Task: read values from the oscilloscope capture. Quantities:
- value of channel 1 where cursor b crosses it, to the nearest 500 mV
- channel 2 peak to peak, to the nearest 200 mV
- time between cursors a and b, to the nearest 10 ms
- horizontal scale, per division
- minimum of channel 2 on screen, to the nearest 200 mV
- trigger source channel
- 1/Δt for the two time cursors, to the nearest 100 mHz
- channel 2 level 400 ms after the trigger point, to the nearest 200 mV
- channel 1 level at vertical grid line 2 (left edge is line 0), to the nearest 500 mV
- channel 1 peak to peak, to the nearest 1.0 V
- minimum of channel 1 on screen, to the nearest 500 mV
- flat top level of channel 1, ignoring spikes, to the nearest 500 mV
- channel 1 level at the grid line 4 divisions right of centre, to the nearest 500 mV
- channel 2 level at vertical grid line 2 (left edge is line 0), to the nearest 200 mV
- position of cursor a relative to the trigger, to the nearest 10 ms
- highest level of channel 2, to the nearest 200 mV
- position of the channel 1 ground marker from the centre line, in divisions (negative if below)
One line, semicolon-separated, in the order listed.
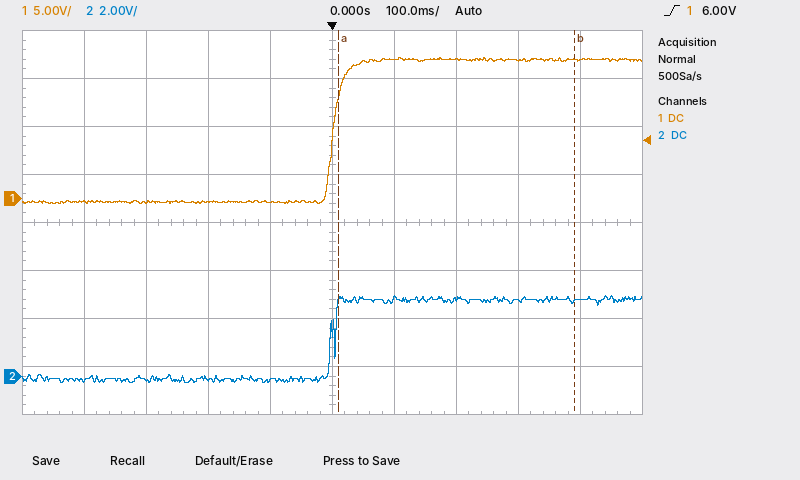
14.5 V; 3.6 V; 380 ms; 100 ms; -200 mV; channel 1; 2.6 Hz; 3.2 V; -500 mV; 15.0 V; -500 mV; 14.5 V; 14.5 V; -200 mV; +10 ms; 3.4 V; +0.5 div
